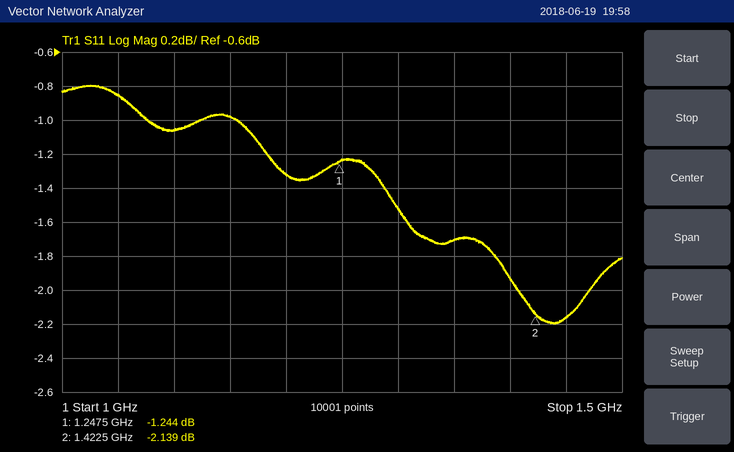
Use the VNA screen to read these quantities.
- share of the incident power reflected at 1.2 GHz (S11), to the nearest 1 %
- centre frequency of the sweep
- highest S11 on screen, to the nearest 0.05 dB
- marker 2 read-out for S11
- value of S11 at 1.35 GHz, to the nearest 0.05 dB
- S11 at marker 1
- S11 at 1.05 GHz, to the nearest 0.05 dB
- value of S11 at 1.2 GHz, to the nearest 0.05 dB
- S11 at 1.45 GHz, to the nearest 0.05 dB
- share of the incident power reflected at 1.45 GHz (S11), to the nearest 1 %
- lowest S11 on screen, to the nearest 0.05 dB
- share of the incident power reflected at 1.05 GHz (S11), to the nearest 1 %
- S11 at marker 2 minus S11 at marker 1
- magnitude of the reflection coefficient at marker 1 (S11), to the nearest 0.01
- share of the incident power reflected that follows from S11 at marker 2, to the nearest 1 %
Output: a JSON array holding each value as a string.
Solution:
["74 %", "1.25 GHz", "-0.80 dB", "-2.139 dB", "-1.70 dB", "-1.244 dB", "-0.85 dB", "-1.30 dB", "-2.15 dB", "61 %", "-2.20 dB", "82 %", "-0.895 dB", "0.87", "61 %"]
